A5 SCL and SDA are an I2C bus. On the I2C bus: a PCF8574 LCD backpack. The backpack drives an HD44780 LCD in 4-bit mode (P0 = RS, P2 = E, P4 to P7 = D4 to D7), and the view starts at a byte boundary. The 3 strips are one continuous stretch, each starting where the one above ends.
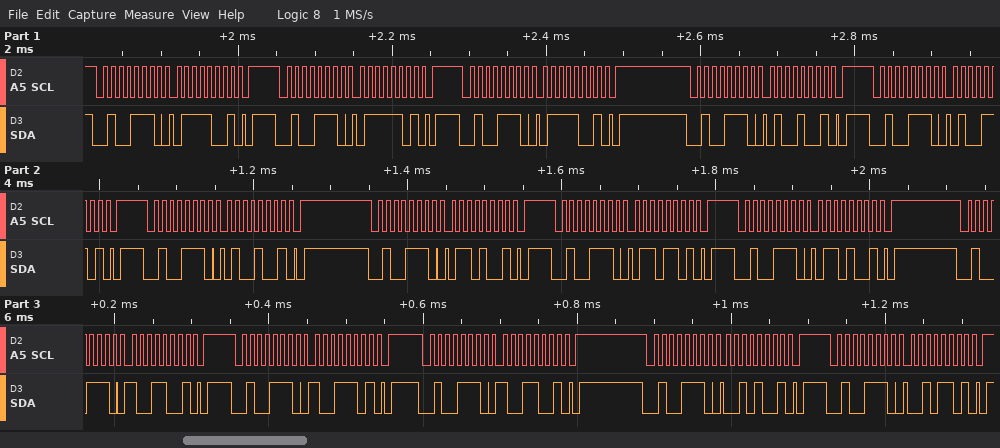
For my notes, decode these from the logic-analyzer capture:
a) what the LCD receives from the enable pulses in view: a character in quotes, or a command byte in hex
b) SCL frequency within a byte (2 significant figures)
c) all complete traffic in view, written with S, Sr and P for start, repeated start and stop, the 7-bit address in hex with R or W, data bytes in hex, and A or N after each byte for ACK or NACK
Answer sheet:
't' 'i'
100 kHz
S 27W A 79 A P S 27W A 7D A P S 27W A 79 A P S 27W A 49 A P S 27W A 4D A P S 27W A 49 A P S 27W A 69 A P S 27W A 6D A P S 27W A 69 A P S 27W A 99 A P S 27W A 9D A P S 27W A 99 A P S 27W A 29 A P S 27W A 2D A P
